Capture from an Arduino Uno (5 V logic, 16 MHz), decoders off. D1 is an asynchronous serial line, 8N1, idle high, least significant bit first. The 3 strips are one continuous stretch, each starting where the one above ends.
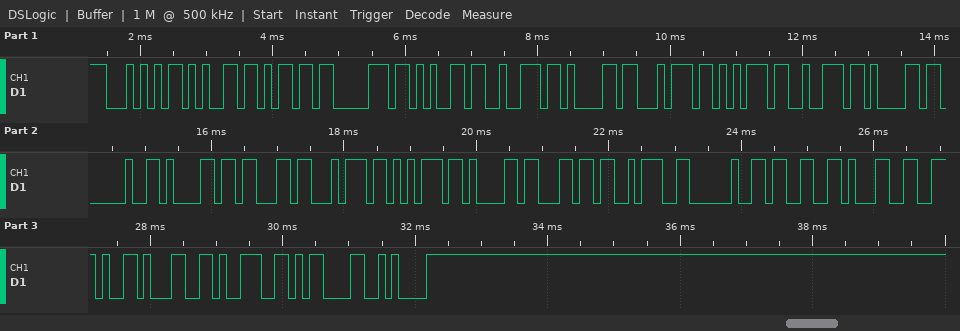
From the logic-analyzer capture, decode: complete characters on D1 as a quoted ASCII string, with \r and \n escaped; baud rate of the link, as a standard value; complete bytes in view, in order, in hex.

"Temperatura actual: 31.19\r\n"
9600 baud
54 65 6D 70 65 72 61 74 75 72 61 20 61 63 74 75 61 6C 3A 20 33 31 2E 31 39 0D 0A
